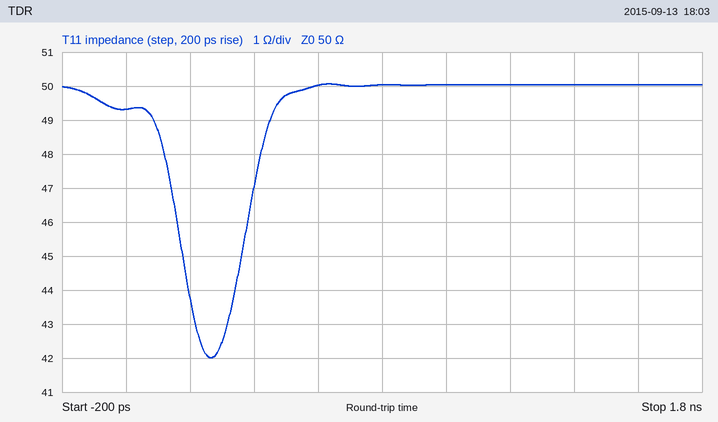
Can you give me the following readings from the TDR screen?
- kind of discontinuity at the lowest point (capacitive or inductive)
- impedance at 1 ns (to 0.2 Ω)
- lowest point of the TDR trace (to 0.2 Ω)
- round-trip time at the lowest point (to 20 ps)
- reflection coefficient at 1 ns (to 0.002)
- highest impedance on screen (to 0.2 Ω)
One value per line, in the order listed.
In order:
capacitive
50.0 Ω
42.0 Ω
260 ps
0.000
50.0 Ω
